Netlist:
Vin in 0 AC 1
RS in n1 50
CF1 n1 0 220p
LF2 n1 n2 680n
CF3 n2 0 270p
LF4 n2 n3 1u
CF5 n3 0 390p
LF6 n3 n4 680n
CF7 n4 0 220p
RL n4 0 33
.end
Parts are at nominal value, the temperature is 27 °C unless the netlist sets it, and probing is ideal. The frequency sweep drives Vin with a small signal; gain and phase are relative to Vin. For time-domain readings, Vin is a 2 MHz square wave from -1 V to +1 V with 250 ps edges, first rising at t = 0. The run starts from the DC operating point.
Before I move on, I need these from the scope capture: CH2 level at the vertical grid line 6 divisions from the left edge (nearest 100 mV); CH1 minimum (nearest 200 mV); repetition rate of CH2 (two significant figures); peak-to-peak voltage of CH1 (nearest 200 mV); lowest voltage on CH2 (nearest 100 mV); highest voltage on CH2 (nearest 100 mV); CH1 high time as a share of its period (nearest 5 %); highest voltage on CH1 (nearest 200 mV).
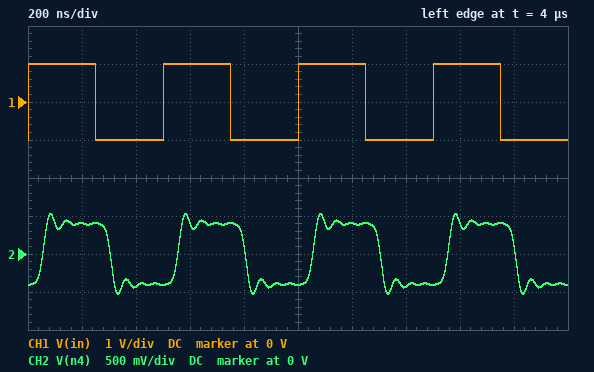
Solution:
400 mV
-1.0 V
2.0 MHz
2.0 V
-500 mV
500 mV
50 %
1.0 V
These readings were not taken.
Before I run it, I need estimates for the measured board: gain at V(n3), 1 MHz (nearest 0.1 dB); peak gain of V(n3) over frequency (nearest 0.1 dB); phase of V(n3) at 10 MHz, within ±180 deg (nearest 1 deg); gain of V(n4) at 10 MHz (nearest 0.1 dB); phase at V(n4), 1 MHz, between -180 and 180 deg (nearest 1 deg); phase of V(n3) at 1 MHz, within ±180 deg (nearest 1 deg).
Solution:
-8.0 dB
-3.3 dB
-116 deg
-8.4 dB
-18 deg
-11 deg
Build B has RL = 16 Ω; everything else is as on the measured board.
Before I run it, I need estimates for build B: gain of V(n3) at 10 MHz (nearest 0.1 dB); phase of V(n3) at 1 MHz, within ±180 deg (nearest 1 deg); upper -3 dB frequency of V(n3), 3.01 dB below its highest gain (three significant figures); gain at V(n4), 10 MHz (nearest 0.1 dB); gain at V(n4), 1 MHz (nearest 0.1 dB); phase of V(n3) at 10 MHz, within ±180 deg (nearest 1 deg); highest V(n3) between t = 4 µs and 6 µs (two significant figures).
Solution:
-3.3 dB
-3 deg
18.1 MHz
-12.0 dB
-12.3 dB
-100 deg
780 mV
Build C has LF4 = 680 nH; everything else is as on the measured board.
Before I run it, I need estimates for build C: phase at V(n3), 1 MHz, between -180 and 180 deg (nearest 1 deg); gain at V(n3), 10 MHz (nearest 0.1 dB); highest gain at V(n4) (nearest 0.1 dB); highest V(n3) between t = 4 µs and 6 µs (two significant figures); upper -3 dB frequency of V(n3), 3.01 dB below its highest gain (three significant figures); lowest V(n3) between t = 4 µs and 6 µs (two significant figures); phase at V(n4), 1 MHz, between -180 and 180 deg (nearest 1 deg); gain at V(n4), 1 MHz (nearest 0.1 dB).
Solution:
-9 deg
-5.3 dB
-7.8 dB
720 mV
20.6 MHz
-720 mV
-17 deg
-8.0 dB
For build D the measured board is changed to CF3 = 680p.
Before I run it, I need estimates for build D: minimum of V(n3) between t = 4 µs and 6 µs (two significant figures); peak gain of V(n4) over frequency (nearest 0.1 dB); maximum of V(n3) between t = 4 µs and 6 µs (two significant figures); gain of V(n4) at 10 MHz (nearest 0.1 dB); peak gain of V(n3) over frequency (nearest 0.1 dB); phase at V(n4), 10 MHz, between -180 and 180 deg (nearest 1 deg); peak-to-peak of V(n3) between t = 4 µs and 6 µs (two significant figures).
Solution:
-600 mV
-7.8 dB
600 mV
-9.7 dB
-5.3 dB
132 deg
1.2 V
